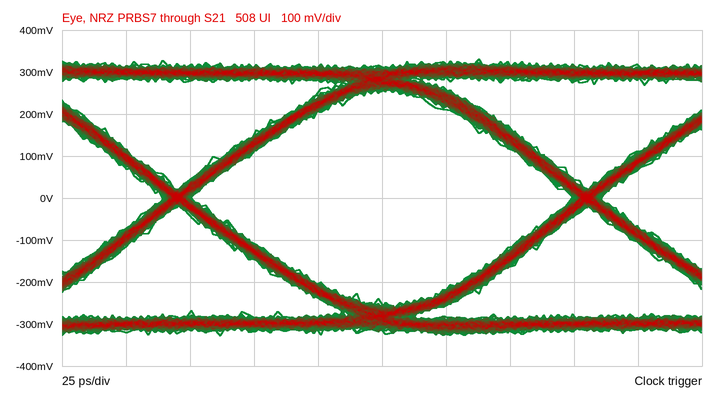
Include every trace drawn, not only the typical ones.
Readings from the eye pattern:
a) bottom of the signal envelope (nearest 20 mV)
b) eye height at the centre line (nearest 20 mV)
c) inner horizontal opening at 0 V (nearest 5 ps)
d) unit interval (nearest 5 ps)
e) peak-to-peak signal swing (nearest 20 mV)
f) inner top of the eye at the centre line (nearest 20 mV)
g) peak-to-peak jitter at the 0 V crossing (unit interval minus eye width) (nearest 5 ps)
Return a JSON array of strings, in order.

["-320 mV", "500 mV", "150 ps", "160 ps", "660 mV", "260 mV", "10 ps"]
